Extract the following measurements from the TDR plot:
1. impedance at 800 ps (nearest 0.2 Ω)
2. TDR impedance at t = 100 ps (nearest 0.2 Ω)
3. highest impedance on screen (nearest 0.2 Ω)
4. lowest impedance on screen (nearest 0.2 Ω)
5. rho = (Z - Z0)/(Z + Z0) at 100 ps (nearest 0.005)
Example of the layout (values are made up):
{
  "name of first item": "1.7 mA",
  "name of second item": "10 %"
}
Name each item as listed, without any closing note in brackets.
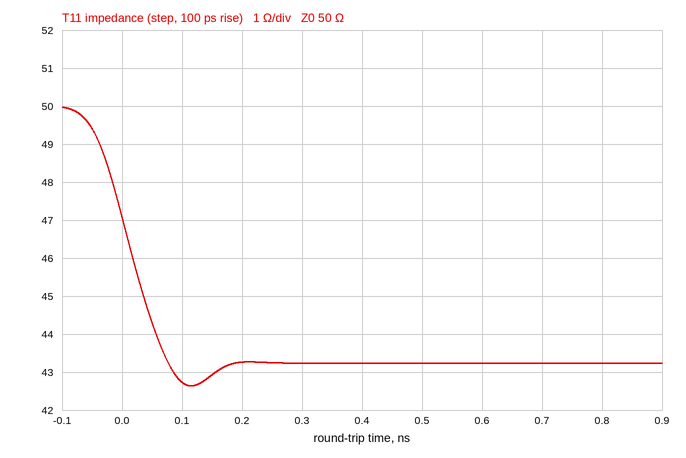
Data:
{
  "impedance at 800 ps": "43.2 Ω",
  "TDR impedance at t = 100 ps": "42.8 Ω",
  "highest impedance on screen": "50.0 Ω",
  "lowest impedance on screen": "42.6 Ω",
  "rho = (Z - Z0)/(Z + Z0) at 100 ps": "-0.080"
}
